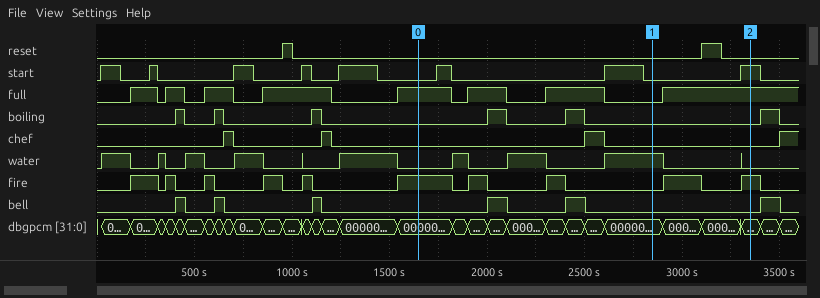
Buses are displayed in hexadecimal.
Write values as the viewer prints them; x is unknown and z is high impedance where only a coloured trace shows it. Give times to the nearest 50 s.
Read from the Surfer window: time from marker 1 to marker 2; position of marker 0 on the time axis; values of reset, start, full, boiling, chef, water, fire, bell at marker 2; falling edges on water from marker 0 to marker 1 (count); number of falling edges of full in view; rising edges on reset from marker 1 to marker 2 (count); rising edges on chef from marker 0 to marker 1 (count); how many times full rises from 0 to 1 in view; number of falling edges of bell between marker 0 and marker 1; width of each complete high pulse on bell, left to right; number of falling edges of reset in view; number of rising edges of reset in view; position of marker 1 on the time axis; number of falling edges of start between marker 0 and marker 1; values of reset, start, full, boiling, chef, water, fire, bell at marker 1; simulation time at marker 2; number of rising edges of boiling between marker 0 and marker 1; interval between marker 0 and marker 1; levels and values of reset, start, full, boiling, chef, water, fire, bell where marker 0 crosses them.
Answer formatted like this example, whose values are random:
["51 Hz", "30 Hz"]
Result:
["500 s", "1650 s", "reset=0, start=1, full=1, boiling=0, chef=0, water=0, fire=1, bell=0", "2", "7", "1", "1", "8", "2", "50 s, 50 s, 50 s, 100 s, 100 s, 100 s", "2", "2", "2850 s", "2", "reset=0, start=0, full=0, boiling=0, chef=0, water=1, fire=0, bell=0", "3350 s", "2", "1200 s", "reset=0, start=0, full=1, boiling=0, chef=0, water=0, fire=1, bell=0"]
